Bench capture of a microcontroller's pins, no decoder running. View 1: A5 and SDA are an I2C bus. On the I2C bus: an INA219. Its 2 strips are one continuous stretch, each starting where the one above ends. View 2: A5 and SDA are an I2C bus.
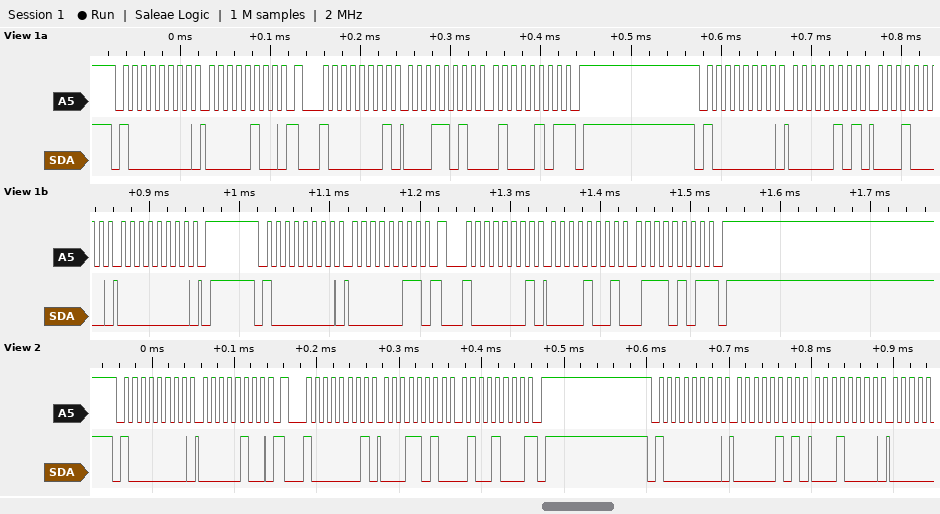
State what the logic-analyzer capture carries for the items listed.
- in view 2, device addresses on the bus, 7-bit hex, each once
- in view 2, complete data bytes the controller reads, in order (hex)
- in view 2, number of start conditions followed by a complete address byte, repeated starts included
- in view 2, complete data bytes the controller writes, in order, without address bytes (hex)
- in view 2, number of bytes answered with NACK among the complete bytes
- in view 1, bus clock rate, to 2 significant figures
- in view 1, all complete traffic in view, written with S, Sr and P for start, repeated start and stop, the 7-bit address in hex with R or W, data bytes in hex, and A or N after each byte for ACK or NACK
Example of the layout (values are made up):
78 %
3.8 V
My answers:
0x40
1A 48
3
04 05 10
1
100 kHz
S 40W A 04 A Sr 40R A 1A A 45 N P S 40W A 05 A 10 A 00 A P S 40W A 03 A Sr 40R A 09 A 75 N P
